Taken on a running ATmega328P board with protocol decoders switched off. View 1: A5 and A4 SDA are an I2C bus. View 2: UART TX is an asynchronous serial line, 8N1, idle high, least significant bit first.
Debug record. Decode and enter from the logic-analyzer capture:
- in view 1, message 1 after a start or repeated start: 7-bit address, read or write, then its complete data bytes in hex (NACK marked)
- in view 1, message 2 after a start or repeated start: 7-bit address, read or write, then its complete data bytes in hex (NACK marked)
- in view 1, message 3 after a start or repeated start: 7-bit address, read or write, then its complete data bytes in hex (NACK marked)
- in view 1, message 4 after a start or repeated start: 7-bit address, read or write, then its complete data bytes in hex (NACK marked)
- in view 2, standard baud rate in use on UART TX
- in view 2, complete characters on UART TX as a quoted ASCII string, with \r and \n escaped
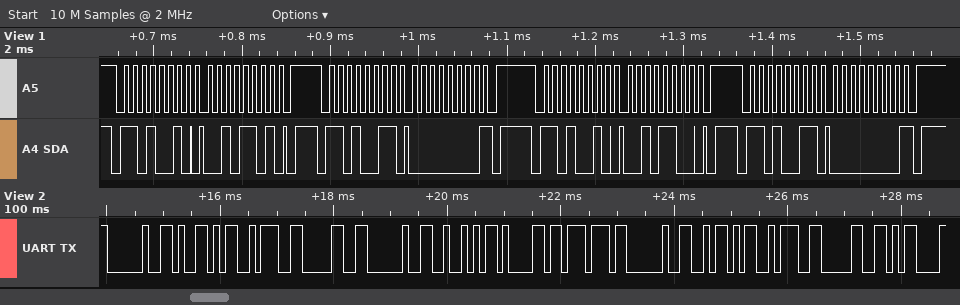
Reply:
0x69 write: 2D
0x69 read: 00 NACK
0x69 write: 2C
0x69 read: 00 NACK
9600 baud
" Y:0 Raw Z:0\r"
